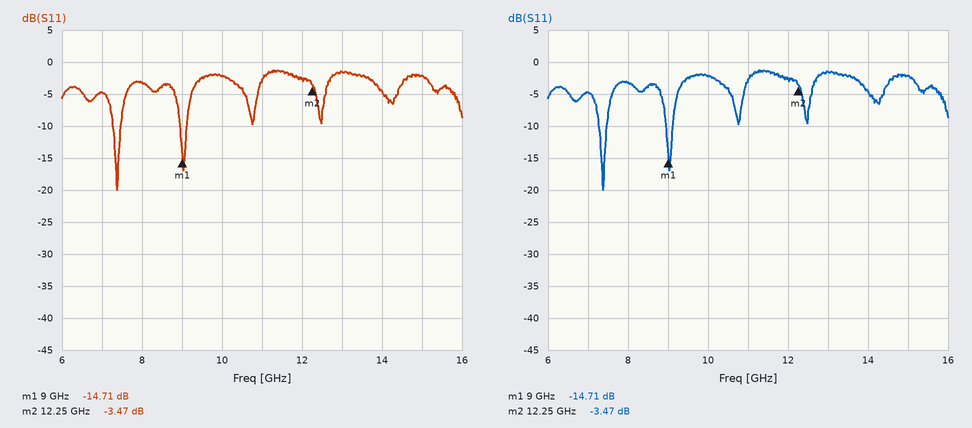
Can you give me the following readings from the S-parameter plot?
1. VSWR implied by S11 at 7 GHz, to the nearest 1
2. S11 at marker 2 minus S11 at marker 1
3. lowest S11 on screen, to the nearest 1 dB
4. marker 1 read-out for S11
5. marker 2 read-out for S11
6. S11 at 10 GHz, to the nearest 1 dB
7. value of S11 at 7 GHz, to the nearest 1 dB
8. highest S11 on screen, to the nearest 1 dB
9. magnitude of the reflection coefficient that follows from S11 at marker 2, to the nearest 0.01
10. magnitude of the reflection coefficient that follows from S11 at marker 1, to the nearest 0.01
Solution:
4
11.24 dB
-20 dB
-14.71 dB
-3.47 dB
-2 dB
-5 dB
-1 dB
0.67
0.18
